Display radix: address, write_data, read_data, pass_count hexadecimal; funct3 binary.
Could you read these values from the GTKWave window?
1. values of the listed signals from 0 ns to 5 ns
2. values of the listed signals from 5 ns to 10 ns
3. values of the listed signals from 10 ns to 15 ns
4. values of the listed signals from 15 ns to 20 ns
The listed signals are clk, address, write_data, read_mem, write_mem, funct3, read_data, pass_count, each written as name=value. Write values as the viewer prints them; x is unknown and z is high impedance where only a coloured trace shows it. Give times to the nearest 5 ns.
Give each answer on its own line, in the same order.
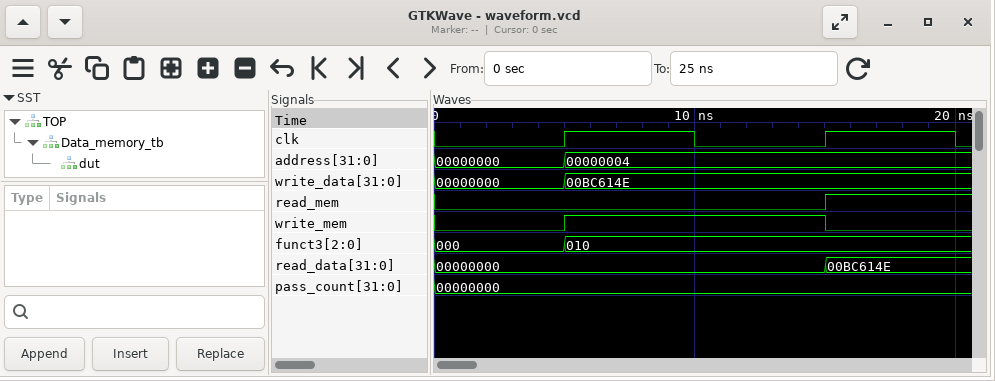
clk=0, address=00000000, write_data=00000000, read_mem=0, write_mem=0, funct3=000, read_data=00000000, pass_count=00000000
clk=1, address=00000004, write_data=00BC614E, read_mem=0, write_mem=1, funct3=010, read_data=00000000, pass_count=00000000
clk=0, address=00000004, write_data=00BC614E, read_mem=0, write_mem=1, funct3=010, read_data=00000000, pass_count=00000000
clk=1, address=00000004, write_data=00BC614E, read_mem=1, write_mem=0, funct3=010, read_data=00BC614E, pass_count=00000000
